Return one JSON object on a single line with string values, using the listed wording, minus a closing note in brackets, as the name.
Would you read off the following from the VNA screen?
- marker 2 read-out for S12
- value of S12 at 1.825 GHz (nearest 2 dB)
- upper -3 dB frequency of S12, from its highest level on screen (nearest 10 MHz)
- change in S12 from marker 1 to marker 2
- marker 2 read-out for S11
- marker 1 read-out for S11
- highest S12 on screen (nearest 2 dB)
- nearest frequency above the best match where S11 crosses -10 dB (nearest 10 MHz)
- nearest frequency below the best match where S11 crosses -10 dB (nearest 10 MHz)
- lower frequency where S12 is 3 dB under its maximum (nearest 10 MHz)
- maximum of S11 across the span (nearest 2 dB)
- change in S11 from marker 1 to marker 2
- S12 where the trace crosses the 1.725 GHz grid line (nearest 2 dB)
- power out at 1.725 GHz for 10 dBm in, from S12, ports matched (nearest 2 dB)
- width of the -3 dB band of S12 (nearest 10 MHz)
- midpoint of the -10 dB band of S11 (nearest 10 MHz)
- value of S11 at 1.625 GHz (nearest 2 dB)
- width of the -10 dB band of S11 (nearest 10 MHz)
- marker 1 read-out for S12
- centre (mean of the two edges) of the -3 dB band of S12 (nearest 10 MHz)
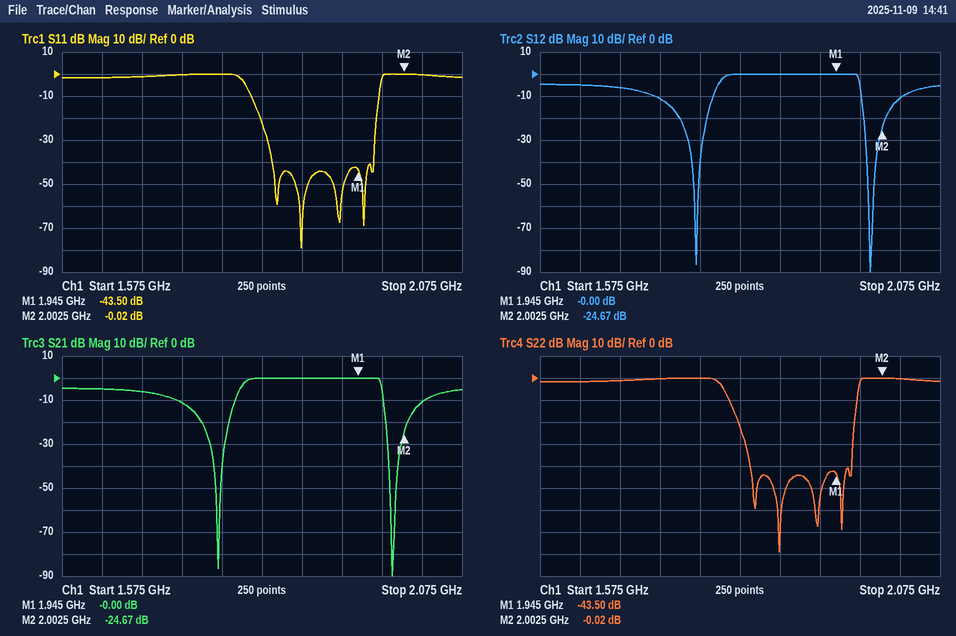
{"marker 2 read-out for S12": "-24.67 dB", "value of S12 at 1.825 GHz": "0 dB", "upper -3 dB frequency of S12, from its highest level on screen": "1.97 GHz", "change in S12 from marker 1 to marker 2": "-24.67 dB", "marker 2 read-out for S11": "-0.02 dB", "marker 1 read-out for S11": "-43.50 dB", "highest S12 on screen": "0 dB", "nearest frequency above the best match where S11 crosses -10 dB": "1.97 GHz", "nearest frequency below the best match where S11 crosses -10 dB": "1.81 GHz", "lower frequency where S12 is 3 dB under its maximum": "1.80 GHz", "maximum of S11 across the span": "0 dB", "change in S11 from marker 1 to marker 2": "43.48 dB", "S12 where the trace crosses the 1.725 GHz grid line": "-12 dB", "power out at 1.725 GHz for 10 dBm in, from S12, ports matched": "-2 dBm", "width of the -3 dB band of S12": "170 MHz", "midpoint of the -10 dB band of S11": "1.89 GHz", "value of S11 at 1.625 GHz": "-2 dB", "width of the -10 dB band of S11": "160 MHz", "marker 1 read-out for S12": "-0.00 dB", "centre (mean of the two edges) of the -3 dB band of S12": "1.89 GHz"}
